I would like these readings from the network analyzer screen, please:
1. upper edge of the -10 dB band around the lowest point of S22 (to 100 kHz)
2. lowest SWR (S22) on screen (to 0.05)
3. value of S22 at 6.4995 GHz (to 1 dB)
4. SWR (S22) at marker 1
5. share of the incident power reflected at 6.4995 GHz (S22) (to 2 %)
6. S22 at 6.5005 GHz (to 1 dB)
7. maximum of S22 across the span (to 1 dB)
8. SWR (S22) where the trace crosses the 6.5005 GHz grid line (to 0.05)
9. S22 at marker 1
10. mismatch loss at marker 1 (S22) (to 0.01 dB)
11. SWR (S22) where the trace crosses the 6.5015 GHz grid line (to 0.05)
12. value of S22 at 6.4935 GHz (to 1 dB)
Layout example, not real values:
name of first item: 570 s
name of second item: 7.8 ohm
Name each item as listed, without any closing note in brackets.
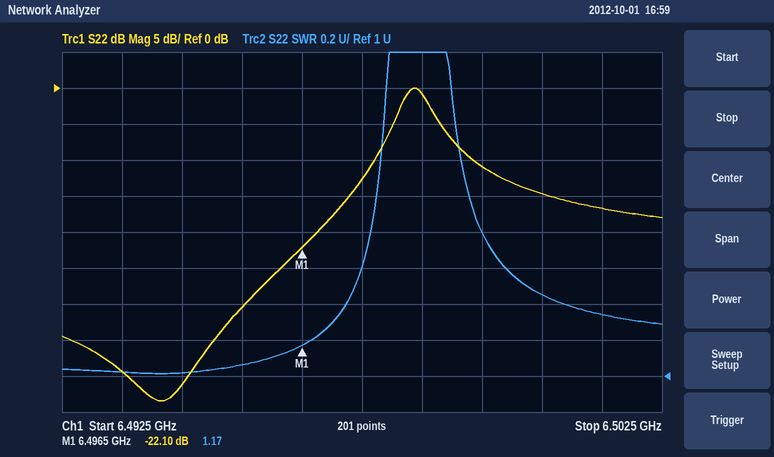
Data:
upper edge of the -10 dB band around the lowest point of S22: 6.4977 GHz
lowest SWR (S22) on screen: 1.00
value of S22 at 6.4995 GHz: -11 dB
SWR (S22) at marker 1: 1.17
share of the incident power reflected at 6.4995 GHz (S22): 8 %
S22 at 6.5005 GHz: -15 dB
maximum of S22 across the span: 0 dB
SWR (S22) where the trace crosses the 6.5005 GHz grid line: 1.45
S22 at marker 1: -22.10 dB
mismatch loss at marker 1 (S22): 0.03 dB
SWR (S22) where the trace crosses the 6.5015 GHz grid line: 1.35
value of S22 at 6.4935 GHz: -39 dB
